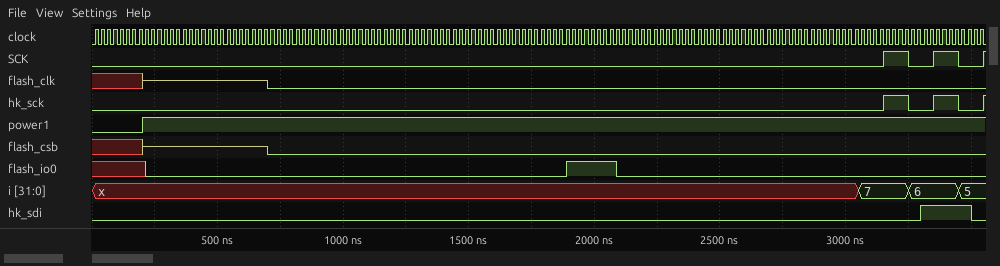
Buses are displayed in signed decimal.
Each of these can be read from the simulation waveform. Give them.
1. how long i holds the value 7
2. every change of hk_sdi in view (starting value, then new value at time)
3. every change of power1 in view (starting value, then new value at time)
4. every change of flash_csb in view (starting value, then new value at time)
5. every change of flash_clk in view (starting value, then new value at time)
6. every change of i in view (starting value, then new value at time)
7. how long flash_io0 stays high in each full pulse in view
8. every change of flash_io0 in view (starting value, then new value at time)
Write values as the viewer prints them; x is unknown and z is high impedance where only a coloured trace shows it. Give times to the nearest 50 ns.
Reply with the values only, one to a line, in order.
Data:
200 ns
0, 1 at 3300 ns, 0 at 3500 ns
0, 1 at 200 ns
x, z at 200 ns, 0 at 700 ns
x, z at 200 ns, 0 at 700 ns
x, 7 at 3050 ns, 6 at 3250 ns, 5 at 3450 ns
200 ns
x, 0 at 200 ns, 1 at 1900 ns, 0 at 2100 ns
